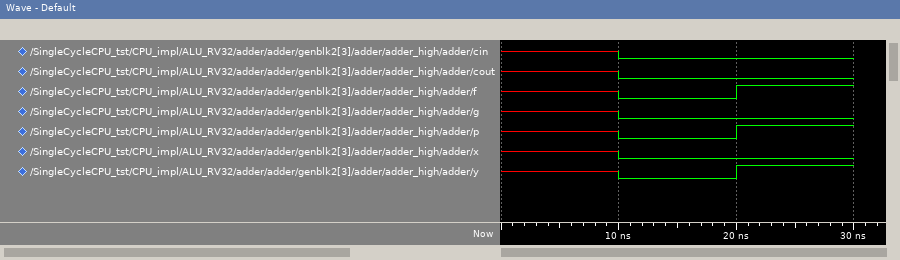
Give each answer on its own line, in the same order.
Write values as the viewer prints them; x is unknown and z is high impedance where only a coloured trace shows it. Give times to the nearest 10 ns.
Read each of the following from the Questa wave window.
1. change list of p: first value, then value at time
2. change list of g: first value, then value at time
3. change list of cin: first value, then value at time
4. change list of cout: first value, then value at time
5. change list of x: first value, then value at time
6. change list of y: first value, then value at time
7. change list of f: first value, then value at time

x, 0 at 10 ns, 1 at 20 ns
x, 0 at 10 ns
x, 0 at 10 ns
x, 0 at 10 ns
x, 0 at 10 ns
x, 0 at 10 ns, 1 at 20 ns
x, 0 at 10 ns, 1 at 20 ns
